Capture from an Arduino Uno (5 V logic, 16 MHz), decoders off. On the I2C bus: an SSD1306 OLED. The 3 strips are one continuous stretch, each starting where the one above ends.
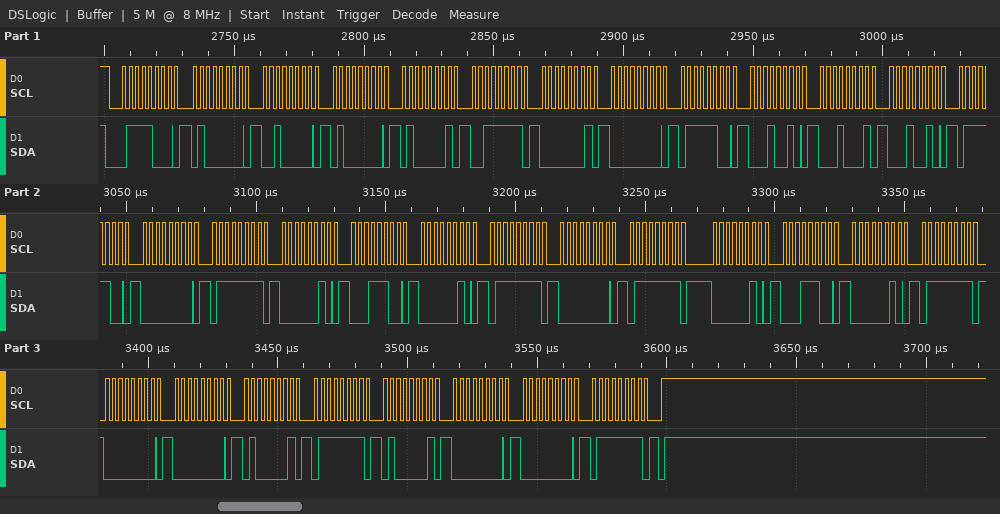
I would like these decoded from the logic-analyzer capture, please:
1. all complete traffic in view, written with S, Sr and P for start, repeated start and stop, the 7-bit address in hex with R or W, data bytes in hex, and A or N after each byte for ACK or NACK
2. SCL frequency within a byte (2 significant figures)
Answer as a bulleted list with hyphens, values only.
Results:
- S 3CW A 40 A 20 A 40 A 41 A 3F A 01 A 00 A 7C A 12 A 11 A 12 A 7C A 00 A 7F A 02 A 1C A 02 A 7F A 00 A 7F A 02 A 1C A 02 A 7F A 00 A 00 A 41 A 7F A 41 A 00 A 00 A 7F A P
- 400 kHz
